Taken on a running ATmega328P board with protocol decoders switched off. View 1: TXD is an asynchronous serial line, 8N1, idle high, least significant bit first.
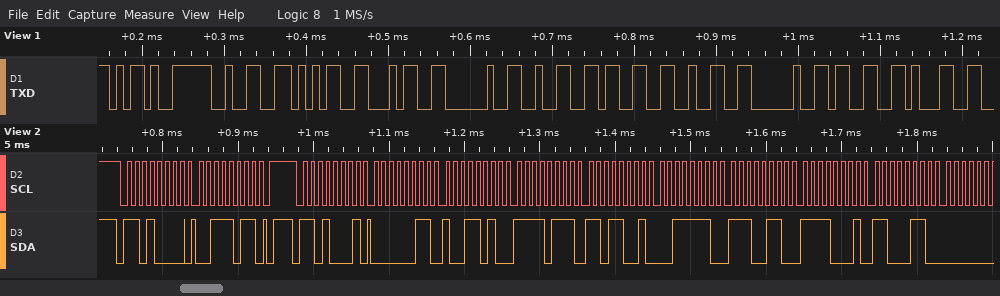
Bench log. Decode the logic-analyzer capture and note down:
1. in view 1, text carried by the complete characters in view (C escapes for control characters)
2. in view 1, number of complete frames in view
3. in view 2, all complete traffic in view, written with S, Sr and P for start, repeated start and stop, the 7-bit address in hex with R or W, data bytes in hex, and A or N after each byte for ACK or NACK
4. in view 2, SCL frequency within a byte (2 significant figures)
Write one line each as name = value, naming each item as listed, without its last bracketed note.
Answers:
in view 1, text carried by the complete characters in view = "-254 232 31"
in view 1, number of complete frames in view = 11
in view 2, all complete traffic in view, written with S, Sr and P for start, repeated start and stop, the 7-bit address in hex with R or W, data bytes in hex, and A or N after each byte for ACK or NACK = S 68W A 3B A P S 68R A 03 A 9A A F7 A D9 A 3E A E6 A F1 A C6 A
in view 2, SCL frequency within a byte = 100 kHz
